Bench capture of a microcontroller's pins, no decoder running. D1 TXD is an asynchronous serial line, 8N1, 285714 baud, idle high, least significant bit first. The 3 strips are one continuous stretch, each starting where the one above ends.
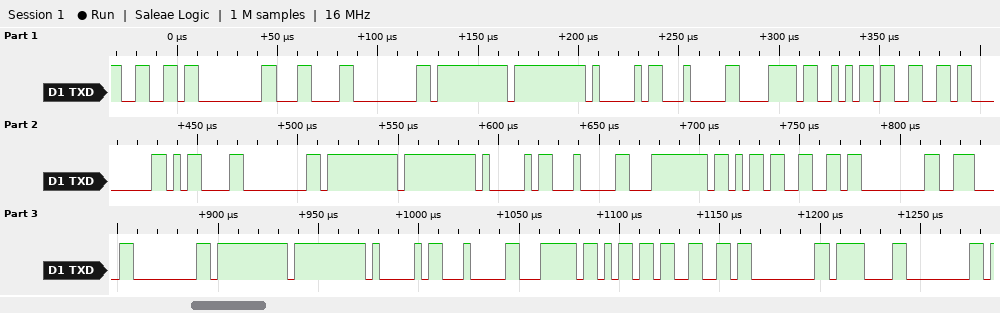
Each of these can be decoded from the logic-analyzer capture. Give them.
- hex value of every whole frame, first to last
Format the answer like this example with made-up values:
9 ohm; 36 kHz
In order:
0x66 0x00 0x0C 0x00 0xFF 0xFF 0x41 0x04 0x78 0x6A 0x66 0x00 0x0D 0x00 0xFF 0xFF 0x41 0x04 0xFC 0x6B 0x66 0x00 0x0E 0x00 0xFF 0xFF 0x41 0x04 0x7C 0x6D 0x66 0x00 0x0F 0x00
